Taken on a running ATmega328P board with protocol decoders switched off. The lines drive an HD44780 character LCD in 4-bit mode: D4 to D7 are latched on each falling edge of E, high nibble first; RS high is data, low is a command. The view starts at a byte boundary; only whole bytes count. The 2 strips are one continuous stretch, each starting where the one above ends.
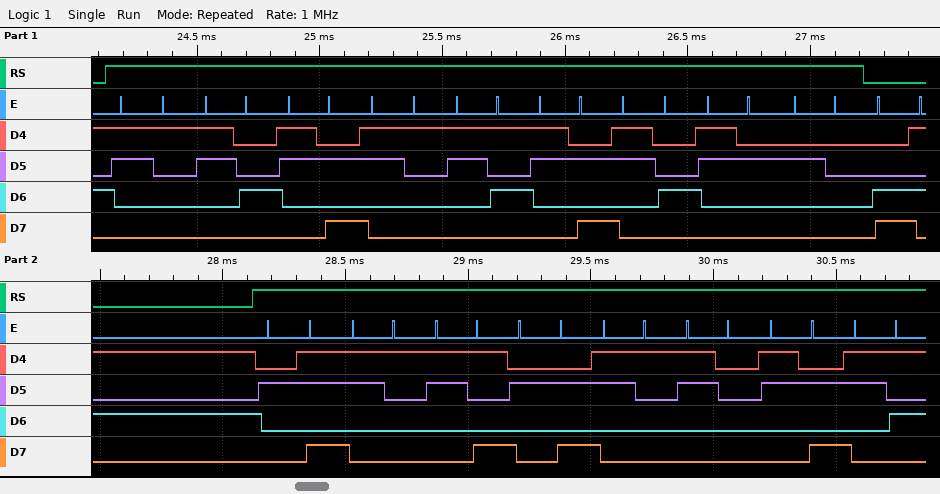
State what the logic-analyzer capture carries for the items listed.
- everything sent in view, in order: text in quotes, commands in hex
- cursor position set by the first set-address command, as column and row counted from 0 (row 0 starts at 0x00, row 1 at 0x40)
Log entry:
"14:15:42 " 0xC5 "+19*10:5"
column 5, row 1
